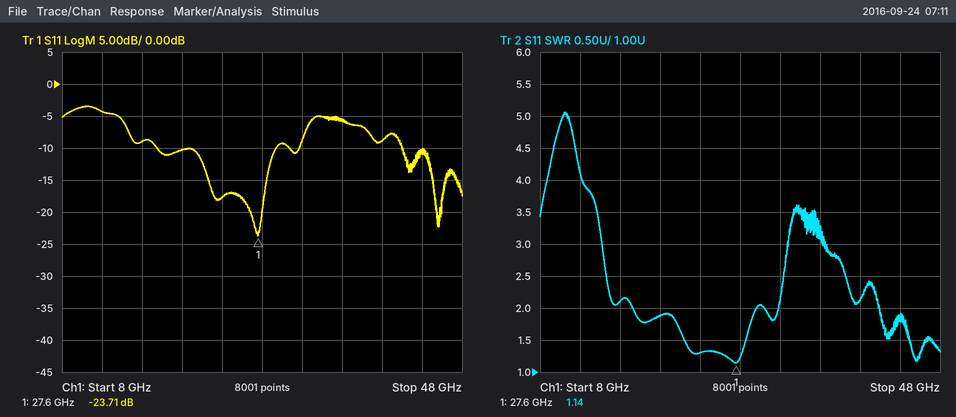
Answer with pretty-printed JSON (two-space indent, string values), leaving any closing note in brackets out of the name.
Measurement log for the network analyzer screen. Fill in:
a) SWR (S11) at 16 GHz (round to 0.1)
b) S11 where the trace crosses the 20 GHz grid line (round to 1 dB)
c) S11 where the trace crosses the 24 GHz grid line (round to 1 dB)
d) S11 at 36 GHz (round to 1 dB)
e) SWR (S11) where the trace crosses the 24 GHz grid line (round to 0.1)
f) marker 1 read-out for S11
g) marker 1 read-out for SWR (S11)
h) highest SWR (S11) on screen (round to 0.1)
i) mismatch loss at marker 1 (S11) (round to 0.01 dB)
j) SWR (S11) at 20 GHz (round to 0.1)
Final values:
{
  "SWR (S11) at 16 GHz": "2.1",
  "S11 where the trace crosses the 20 GHz grid line": "-10 dB",
  "S11 where the trace crosses the 24 GHz grid line": "-18 dB",
  "S11 at 36 GHz": "-6 dB",
  "SWR (S11) where the trace crosses the 24 GHz grid line": "1.3",
  "marker 1 read-out for S11": "-23.71 dB",
  "marker 1 read-out for SWR": "1.14",
  "highest SWR (S11) on screen": "5.1",
  "mismatch loss at marker 1 (S11)": "0.02 dB",
  "SWR (S11) at 20 GHz": "1.9"
}
